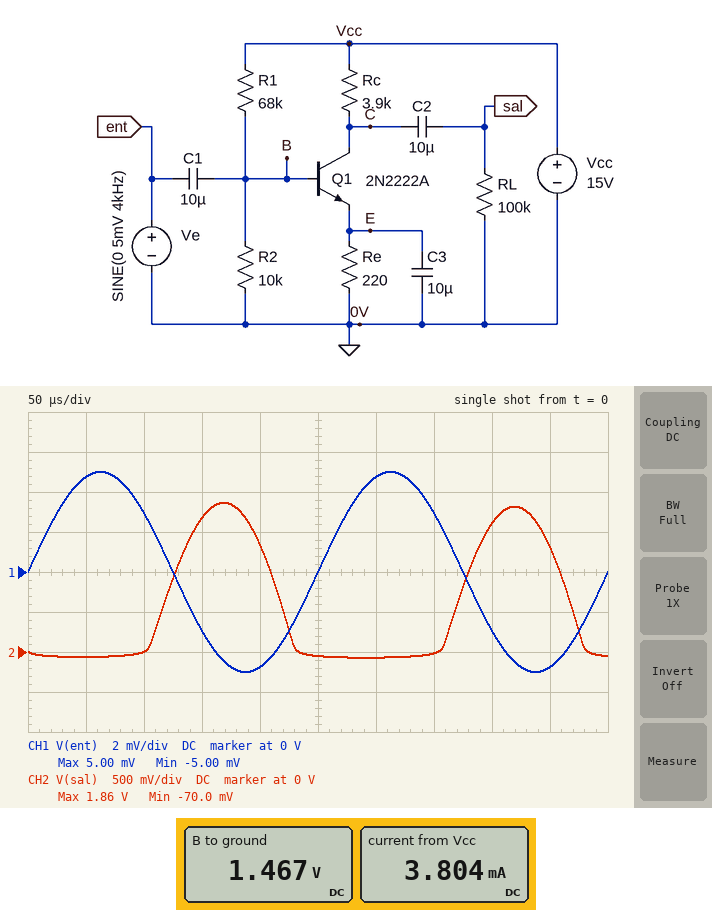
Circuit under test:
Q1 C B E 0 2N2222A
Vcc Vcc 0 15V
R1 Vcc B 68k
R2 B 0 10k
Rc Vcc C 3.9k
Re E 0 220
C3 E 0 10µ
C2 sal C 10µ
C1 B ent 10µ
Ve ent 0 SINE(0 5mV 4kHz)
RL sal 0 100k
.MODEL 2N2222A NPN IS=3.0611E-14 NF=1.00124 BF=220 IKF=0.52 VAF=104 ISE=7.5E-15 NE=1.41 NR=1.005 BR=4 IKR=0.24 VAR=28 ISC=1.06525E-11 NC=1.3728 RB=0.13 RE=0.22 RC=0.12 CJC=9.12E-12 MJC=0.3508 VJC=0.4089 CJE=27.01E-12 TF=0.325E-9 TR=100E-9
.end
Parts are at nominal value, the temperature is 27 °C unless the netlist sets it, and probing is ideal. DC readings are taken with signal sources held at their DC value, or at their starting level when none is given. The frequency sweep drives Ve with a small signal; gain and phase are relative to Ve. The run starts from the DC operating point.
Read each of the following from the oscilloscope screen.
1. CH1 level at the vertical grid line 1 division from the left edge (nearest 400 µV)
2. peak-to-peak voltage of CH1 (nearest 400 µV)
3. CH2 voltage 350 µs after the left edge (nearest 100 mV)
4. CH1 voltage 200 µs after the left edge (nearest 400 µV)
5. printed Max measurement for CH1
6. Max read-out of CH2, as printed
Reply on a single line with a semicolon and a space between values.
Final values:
4.8 mV; 10.0 mV; 0 V; -4.8 mV; 5.00 mV; 1.86 V
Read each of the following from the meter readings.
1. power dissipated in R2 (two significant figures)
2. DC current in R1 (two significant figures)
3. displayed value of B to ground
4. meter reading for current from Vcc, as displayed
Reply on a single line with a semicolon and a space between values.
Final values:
220 µW; 200 µA; 1.467 V; 3.804 mA
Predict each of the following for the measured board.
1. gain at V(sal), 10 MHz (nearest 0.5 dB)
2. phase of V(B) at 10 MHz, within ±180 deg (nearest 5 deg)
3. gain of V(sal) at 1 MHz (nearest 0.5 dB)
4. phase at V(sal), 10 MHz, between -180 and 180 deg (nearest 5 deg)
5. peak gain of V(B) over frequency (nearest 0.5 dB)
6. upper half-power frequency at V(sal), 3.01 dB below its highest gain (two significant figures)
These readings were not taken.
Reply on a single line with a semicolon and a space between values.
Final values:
26.5 dB; 0 deg; 36.0 dB; 105 deg; 0 dB; 3.5 MHz
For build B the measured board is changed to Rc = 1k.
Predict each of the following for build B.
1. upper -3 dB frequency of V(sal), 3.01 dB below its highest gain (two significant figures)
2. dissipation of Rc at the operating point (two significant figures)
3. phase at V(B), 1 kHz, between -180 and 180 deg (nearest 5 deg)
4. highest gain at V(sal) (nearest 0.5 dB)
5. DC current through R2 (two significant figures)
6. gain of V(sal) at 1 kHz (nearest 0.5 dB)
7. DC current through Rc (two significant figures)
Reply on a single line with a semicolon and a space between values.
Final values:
53 MHz; 23 mW; 0 deg; 44.5 dB; 170 µA; 35.0 dB; 4.8 mA
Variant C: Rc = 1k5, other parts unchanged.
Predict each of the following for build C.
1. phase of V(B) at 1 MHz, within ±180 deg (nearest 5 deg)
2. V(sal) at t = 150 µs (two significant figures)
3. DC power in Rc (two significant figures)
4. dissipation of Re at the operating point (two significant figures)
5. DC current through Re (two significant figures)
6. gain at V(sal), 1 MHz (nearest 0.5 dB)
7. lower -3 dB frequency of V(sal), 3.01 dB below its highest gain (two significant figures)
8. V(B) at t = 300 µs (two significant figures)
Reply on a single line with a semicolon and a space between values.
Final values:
0 deg; 950 mV; 35 mW; 5.1 mW; 4.8 mA; 48.0 dB; 2.7 kHz; 1.7 V
